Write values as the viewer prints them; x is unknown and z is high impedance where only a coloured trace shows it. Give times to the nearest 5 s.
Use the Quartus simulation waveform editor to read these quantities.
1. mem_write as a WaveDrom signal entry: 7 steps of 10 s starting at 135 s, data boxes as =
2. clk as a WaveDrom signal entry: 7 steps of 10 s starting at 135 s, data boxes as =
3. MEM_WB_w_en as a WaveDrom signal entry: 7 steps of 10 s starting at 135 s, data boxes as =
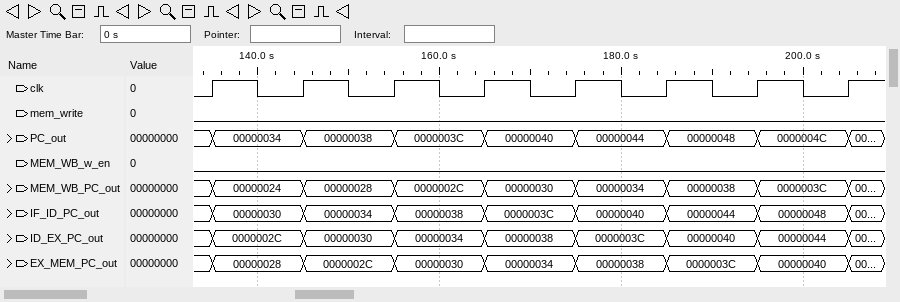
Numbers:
{name: 'mem_write', wave: '0......'}
{name: 'clk', wave: 'p......'}
{name: 'MEM_WB_w_en', wave: '0......'}
